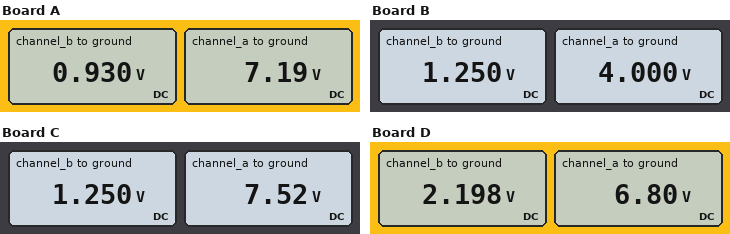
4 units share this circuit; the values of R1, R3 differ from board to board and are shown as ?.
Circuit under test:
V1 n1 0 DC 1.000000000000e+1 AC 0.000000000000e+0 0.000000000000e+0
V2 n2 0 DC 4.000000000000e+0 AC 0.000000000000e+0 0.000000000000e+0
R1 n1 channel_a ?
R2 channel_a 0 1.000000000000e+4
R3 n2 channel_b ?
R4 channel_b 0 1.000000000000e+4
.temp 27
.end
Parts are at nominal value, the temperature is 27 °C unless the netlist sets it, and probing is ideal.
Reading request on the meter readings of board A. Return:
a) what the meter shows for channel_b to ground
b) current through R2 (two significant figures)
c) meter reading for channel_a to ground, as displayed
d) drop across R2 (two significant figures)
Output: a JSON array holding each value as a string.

["0.930 V", "720 µA", "7.19 V", "7.2 V"]
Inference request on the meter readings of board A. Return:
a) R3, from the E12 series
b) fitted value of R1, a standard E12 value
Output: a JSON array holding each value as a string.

["33 kΩ", "3.9 kΩ"]
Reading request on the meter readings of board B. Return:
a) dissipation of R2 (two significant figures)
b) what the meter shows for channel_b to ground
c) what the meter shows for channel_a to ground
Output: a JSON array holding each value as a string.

["1.6 mW", "1.250 V", "4.000 V"]
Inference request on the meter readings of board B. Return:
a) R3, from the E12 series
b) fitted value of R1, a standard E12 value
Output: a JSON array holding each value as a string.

["22 kΩ", "15 kΩ"]
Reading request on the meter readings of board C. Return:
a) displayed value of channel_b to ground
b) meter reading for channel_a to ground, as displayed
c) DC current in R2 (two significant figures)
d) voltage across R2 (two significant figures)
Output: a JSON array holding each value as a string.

["1.250 V", "7.52 V", "750 µA", "7.5 V"]
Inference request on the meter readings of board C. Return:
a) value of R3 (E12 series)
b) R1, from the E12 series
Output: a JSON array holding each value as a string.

["22 kΩ", "3.3 kΩ"]
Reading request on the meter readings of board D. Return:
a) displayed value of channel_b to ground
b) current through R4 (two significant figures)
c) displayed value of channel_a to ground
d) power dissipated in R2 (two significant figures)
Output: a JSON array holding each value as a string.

["2.198 V", "220 µA", "6.80 V", "4.6 mW"]
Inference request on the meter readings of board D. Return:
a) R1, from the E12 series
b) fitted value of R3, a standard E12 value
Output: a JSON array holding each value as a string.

["4.7 kΩ", "8.2 kΩ"]
